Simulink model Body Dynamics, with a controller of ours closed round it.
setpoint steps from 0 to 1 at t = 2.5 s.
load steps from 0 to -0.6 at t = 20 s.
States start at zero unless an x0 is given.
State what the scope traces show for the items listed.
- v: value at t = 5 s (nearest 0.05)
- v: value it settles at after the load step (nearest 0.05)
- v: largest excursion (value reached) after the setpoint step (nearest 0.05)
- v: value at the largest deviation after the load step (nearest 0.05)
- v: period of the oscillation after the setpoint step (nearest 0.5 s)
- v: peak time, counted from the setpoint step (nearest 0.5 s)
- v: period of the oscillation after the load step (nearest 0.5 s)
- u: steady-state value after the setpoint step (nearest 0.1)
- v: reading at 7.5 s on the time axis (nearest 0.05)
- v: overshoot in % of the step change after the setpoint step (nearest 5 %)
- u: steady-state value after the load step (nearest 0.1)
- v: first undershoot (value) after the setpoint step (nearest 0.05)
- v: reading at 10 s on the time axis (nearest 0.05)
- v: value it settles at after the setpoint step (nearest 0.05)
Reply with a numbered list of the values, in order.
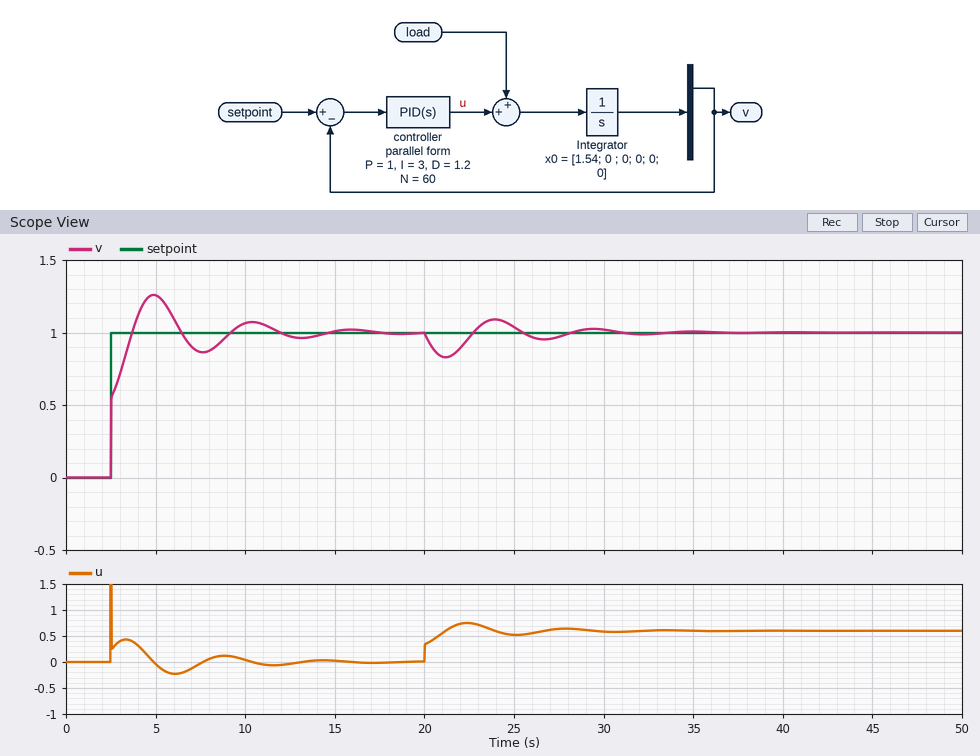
1. 1.25
2. 1.00
3. 1.25
4. 0.85
5. 5.5 s
6. 2.5 s
7. 5.5 s
8. 0.0
9. 0.85
10. 25 %
11. 0.6
12. 0.85
13. 1.05
14. 1.00
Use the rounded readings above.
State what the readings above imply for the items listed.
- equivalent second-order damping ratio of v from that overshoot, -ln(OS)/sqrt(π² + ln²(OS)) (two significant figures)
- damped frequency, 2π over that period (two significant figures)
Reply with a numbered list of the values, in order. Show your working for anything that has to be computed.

1. ln(0.25) = -1.386; 1.386 / sqrt(9.870 + 1.922) = 0.40
2. 2π / 5.5 = 1.1 rad/s
